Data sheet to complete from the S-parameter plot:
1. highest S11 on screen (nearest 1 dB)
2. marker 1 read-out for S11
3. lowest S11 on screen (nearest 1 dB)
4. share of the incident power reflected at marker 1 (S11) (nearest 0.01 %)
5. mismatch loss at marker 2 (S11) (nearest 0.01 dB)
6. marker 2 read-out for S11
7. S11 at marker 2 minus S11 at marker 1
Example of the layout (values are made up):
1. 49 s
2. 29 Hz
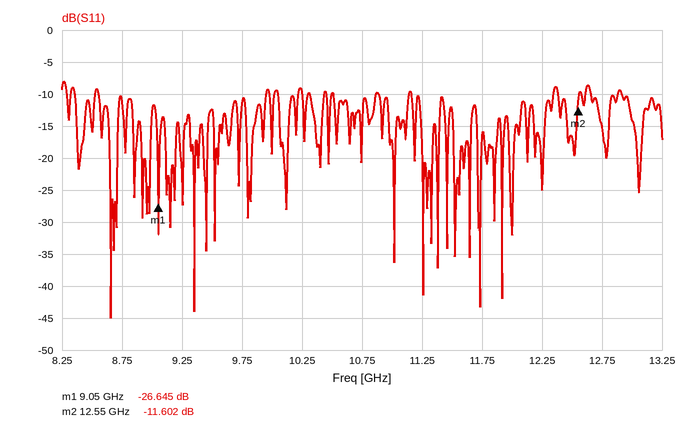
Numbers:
1. -8 dB
2. -26.645 dB
3. -45 dB
4. 0.22 %
5. 0.31 dB
6. -11.602 dB
7. 15.043 dB
